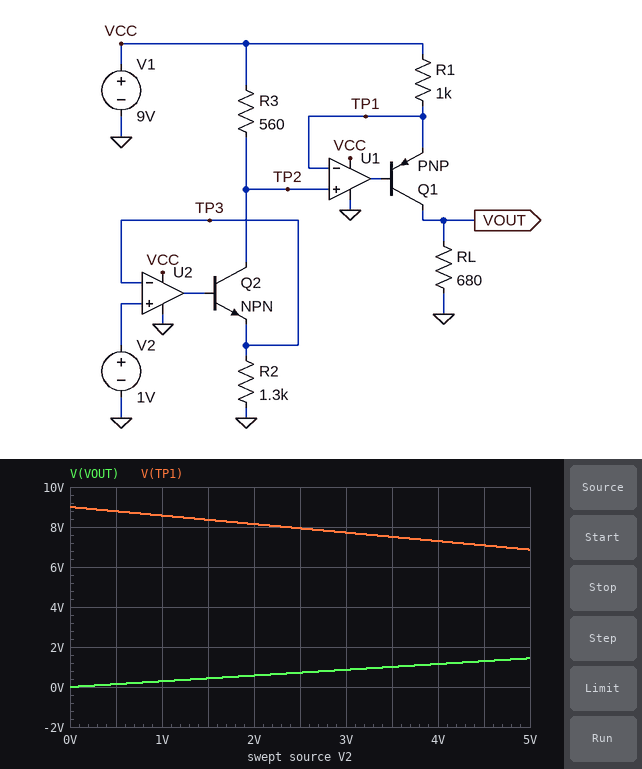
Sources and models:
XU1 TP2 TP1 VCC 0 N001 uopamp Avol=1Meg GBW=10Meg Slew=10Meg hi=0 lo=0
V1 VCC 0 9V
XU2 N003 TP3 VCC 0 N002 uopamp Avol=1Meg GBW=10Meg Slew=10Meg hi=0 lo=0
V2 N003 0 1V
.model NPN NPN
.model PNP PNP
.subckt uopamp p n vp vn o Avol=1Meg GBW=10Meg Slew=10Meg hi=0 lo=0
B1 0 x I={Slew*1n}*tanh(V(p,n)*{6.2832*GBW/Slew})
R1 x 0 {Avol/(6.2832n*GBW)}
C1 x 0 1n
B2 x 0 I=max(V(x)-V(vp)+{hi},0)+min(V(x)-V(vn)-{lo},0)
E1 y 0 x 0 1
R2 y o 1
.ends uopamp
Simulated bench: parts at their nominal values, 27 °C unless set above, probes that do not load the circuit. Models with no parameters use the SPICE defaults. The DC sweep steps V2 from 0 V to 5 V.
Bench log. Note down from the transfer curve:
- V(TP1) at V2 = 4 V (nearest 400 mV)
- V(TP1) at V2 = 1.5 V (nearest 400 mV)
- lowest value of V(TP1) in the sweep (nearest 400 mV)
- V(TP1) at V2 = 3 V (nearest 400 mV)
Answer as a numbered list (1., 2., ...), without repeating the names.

1. 7.2 V
2. 8.4 V
3. 6.8 V
4. 7.6 V
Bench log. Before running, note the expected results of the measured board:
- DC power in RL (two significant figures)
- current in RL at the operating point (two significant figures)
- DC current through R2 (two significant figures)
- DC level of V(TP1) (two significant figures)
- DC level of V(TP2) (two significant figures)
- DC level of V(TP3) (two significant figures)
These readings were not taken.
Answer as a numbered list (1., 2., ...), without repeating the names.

1. 120 µW
2. 420 µA
3. 770 µA
4. 8.6 V
5. 8.6 V
6. 1.0 V
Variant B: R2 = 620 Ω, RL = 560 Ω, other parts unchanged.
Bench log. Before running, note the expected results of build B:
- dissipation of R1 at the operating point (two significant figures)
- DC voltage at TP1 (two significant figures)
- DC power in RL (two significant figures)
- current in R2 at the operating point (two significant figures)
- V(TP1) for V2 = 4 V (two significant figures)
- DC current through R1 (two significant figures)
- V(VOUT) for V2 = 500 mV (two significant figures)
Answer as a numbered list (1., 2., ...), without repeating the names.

1. 800 µW
2. 8.1 V
3. 440 µW
4. 1.6 mA
5. 5.4 V
6. 890 µA
7. 250 mV
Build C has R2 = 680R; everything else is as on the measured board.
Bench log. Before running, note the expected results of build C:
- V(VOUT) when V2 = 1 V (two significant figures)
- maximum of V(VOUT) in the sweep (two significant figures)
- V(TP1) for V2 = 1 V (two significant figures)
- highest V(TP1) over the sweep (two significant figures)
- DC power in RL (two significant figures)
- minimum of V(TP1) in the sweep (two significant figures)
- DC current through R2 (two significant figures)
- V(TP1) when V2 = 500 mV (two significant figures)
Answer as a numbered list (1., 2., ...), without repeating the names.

1. 550 mV
2. 2.7 V
3. 8.2 V
4. 9.0 V
5. 440 µW
6. 5.0 V
7. 1.5 mA
8. 8.6 V
